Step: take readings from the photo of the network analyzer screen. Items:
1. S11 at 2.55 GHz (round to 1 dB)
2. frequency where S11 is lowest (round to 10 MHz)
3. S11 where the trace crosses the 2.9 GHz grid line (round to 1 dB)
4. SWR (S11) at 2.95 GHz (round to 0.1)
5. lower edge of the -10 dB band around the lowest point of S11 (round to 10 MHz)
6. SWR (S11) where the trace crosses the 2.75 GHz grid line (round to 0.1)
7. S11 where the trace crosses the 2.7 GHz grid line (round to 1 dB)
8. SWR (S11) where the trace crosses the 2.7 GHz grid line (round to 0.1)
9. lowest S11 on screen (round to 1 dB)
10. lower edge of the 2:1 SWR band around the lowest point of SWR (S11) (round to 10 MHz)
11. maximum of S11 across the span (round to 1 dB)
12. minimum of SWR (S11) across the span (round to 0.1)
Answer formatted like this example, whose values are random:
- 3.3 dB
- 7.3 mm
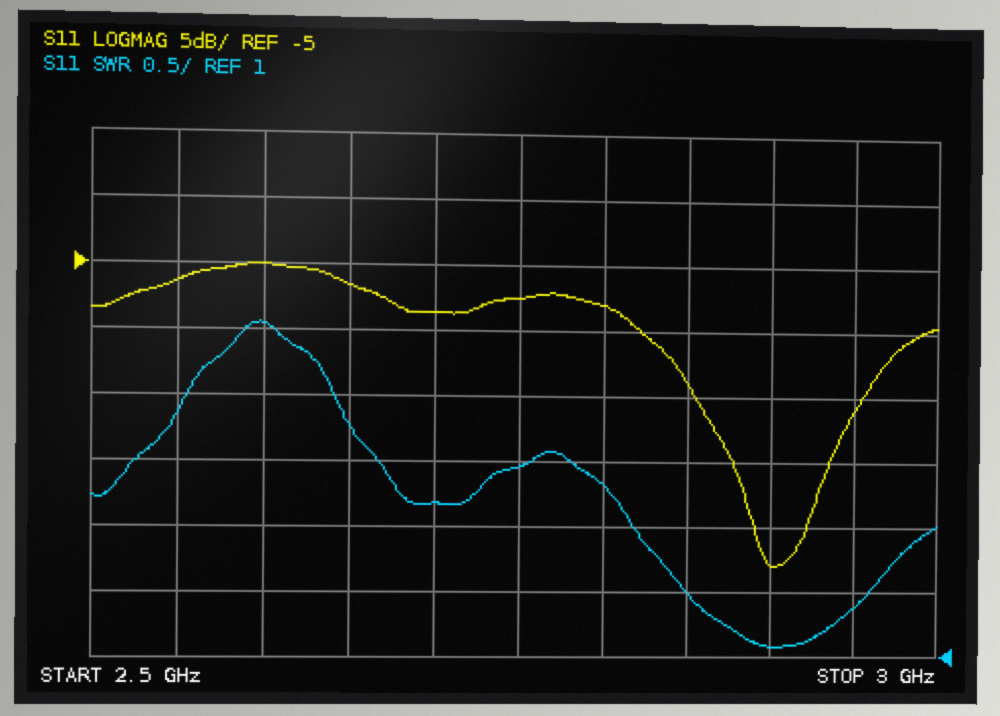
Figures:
- -6 dB
- 2.90 GHz
- -28 dB
- 1.4
- 2.82 GHz
- 2.5
- -9 dB
- 2.2
- -28 dB
- 2.82 GHz
- -5 dB
- 1.1
